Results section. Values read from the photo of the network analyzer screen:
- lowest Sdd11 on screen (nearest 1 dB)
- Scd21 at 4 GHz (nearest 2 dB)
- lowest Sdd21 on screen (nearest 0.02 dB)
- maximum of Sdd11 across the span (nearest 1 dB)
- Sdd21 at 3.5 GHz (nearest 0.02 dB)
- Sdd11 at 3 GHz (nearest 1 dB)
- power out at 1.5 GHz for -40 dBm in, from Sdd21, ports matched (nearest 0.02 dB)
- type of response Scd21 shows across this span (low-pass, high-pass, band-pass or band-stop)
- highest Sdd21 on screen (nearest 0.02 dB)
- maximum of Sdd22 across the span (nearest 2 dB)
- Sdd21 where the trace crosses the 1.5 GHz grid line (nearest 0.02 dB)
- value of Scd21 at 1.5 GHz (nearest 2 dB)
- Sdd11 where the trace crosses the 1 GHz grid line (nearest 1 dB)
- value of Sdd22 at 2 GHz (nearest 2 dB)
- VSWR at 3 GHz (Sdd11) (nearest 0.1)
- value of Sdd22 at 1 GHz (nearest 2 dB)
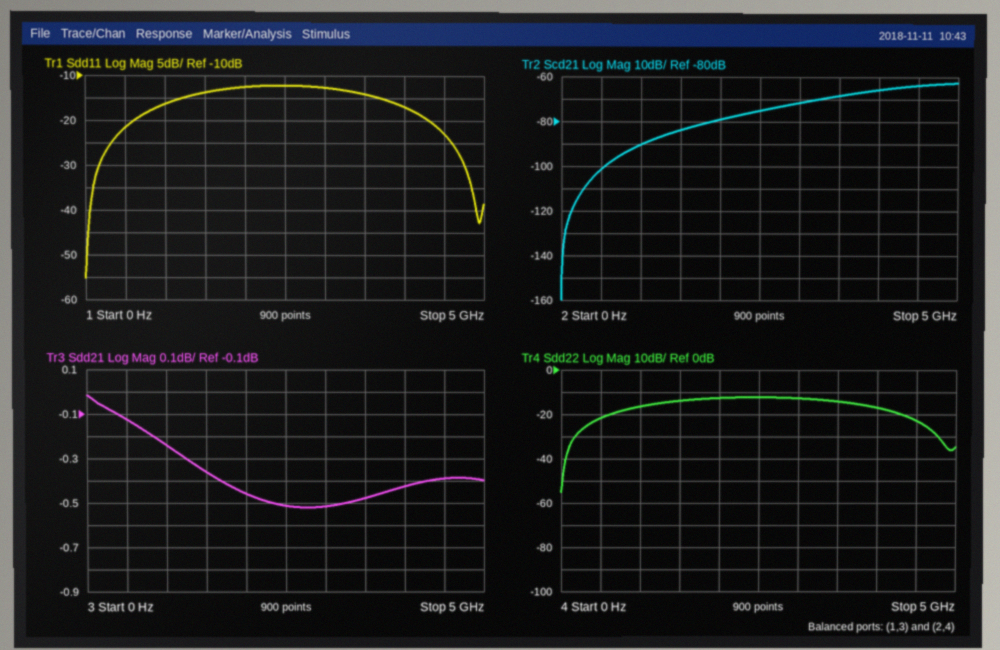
-55 dB
-66 dB
-0.52 dB
-12 dB
-0.48 dB
-13 dB
-40.36 dBm
high-pass
-0.02 dB
-12 dB
-0.36 dB
-84 dB
-16 dB
-12 dB
1.6
-16 dB
